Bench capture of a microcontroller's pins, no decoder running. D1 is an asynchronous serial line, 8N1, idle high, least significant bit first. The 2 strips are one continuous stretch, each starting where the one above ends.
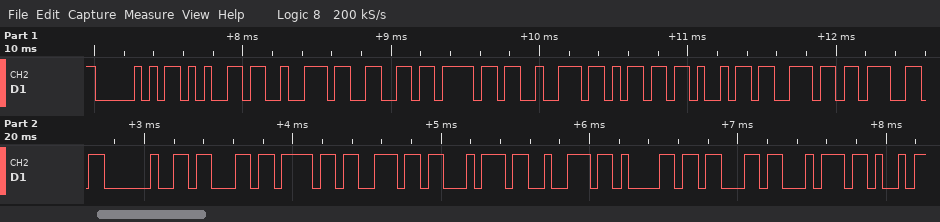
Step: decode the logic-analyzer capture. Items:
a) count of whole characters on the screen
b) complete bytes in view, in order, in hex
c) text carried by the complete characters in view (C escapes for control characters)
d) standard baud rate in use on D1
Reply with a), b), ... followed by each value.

a) 19
b) 0x50 0x65 0x72 0x66 0x6F 0x72 0x6D 0x69 0x6E 0x67 0x20 0x63 0x6F 0x6E 0x74 0x72 0x61 0x63 0x74
c) "Performing contract"
d) 19200 baud
